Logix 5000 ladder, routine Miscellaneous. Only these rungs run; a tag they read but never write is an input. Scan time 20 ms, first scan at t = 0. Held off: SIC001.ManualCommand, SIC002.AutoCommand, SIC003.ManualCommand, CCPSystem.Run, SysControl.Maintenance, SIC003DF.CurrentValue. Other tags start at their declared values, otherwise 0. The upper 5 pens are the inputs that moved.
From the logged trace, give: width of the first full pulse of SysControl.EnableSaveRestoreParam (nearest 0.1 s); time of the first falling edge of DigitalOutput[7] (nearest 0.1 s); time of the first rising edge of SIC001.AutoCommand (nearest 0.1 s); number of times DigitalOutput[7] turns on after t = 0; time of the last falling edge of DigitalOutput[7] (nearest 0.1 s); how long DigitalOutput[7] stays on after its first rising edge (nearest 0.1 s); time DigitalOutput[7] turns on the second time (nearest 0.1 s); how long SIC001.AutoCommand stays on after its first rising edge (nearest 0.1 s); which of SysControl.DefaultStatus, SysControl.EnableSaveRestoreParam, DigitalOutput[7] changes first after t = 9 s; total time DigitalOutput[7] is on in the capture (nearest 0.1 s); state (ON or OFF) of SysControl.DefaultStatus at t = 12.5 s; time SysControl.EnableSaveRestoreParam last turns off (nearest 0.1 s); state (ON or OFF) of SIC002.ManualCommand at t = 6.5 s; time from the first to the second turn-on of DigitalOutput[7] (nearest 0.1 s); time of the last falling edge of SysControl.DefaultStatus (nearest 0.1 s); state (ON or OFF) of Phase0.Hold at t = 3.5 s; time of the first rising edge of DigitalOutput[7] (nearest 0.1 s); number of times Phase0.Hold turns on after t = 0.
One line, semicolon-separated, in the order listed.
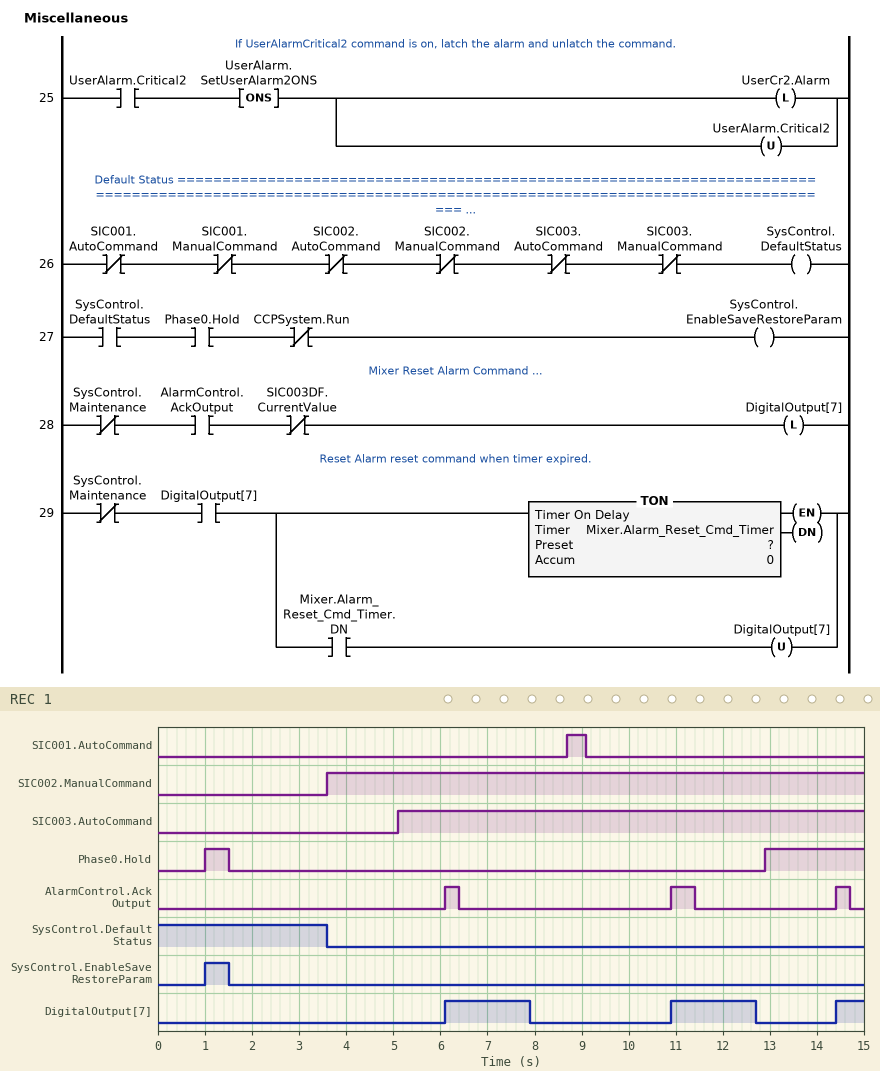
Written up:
0.5 s; 7.9 s; 8.7 s; 3; 12.7 s; 1.8 s; 10.9 s; 0.4 s; DigitalOutput[7]; 4.2 s; OFF; 1.5 s; ON; 4.8 s; 3.6 s; OFF; 6.1 s; 2
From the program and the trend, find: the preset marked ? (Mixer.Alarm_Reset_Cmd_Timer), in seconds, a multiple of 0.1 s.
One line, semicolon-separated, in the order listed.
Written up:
1.8 s
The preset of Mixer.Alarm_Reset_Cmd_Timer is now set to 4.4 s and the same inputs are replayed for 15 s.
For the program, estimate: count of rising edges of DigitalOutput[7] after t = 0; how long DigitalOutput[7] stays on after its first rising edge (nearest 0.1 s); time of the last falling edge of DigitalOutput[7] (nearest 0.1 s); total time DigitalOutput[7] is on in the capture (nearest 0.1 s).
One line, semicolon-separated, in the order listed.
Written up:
2; 4.4 s; 10.5 s; 8.5 s
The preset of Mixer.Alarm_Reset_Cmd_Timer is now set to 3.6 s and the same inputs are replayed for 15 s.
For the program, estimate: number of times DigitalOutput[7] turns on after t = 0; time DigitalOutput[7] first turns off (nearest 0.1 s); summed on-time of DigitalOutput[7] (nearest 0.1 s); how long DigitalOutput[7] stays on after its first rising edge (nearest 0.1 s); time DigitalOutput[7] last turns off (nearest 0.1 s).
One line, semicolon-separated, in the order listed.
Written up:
2; 9.7 s; 7.2 s; 3.6 s; 14.5 s
